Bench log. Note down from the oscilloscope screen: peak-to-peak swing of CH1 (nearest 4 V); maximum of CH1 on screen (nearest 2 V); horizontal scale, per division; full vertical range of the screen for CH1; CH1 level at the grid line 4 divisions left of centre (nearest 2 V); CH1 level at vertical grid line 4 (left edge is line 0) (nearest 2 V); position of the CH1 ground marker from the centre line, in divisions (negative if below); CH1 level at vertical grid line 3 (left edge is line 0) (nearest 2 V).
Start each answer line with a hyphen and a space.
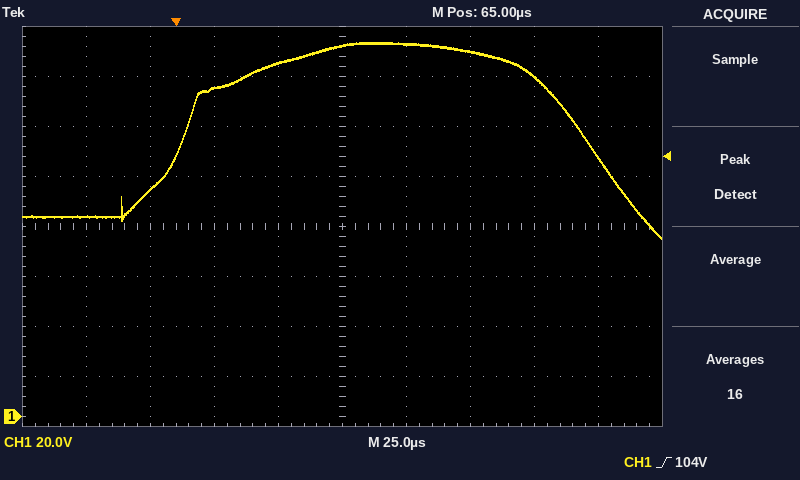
- 80 V
- 150 V
- 25 µs
- 160 V
- 80 V
- 142 V
- -3.8 div
- 132 V
